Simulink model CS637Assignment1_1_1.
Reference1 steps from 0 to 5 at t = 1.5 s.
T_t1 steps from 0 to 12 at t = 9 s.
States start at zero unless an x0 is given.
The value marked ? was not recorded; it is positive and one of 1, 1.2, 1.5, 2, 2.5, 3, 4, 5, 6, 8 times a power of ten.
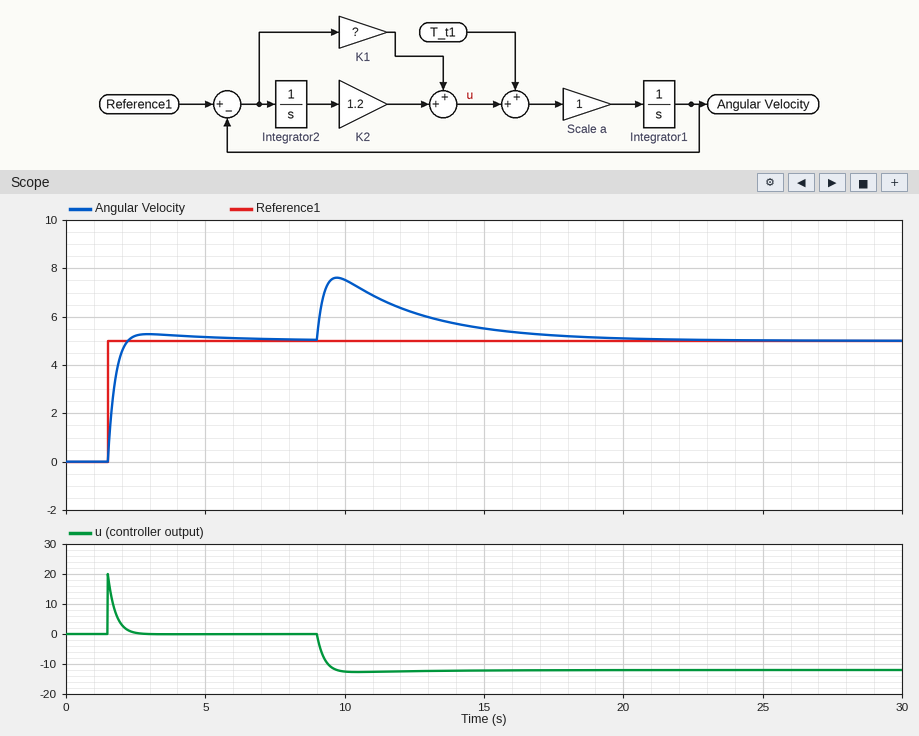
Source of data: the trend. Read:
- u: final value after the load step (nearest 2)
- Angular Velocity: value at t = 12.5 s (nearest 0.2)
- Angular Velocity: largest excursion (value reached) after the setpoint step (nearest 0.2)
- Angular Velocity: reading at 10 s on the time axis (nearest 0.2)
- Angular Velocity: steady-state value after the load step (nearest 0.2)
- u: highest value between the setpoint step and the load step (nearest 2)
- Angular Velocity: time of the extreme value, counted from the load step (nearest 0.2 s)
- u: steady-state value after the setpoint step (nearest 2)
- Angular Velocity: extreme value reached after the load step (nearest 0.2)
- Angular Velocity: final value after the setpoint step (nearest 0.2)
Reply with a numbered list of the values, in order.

1. -12
2. 6.2
3. 5.2
4. 7.6
5. 5.0
6. 20
7. 0.8 s
8. 0
9. 7.6
10. 5.0
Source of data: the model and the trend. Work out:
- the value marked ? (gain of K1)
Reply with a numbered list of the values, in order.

1. 4
